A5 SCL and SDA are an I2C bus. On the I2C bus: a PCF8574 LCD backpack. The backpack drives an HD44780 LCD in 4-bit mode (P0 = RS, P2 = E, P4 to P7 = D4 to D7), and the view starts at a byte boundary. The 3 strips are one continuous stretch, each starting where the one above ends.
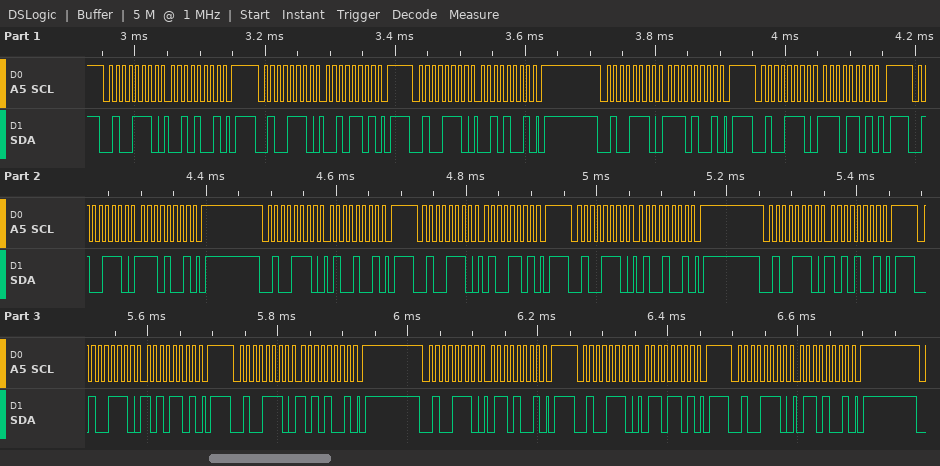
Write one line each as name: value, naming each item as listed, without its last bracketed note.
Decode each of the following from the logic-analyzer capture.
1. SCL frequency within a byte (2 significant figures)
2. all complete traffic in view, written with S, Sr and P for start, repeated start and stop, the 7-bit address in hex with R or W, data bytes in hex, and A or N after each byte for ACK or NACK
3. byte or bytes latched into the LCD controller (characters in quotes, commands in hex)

SCL frequency within a byte: 100 kHz
all complete traffic in view, written with S, Sr and P for start, repeated start and stop, the 7-bit address in hex with R or W, data bytes in hex, and A or N after each byte for ACK or NACK: S 27W A 29 A P S 27W A 2D A P S 27W A 29 A P S 27W A E9 A P S 27W A ED A P S 27W A E9 A P S 27W A 49 A P S 27W A 4D A P S 27W A 49 A P S 27W A A9 A P S 27W A AD A P S 27W A A9 A P S 27W A 69 A P S 27W A 6D A P S 27W A 69 A P
byte or bytes latched into the LCD controller: '.' 'J'
